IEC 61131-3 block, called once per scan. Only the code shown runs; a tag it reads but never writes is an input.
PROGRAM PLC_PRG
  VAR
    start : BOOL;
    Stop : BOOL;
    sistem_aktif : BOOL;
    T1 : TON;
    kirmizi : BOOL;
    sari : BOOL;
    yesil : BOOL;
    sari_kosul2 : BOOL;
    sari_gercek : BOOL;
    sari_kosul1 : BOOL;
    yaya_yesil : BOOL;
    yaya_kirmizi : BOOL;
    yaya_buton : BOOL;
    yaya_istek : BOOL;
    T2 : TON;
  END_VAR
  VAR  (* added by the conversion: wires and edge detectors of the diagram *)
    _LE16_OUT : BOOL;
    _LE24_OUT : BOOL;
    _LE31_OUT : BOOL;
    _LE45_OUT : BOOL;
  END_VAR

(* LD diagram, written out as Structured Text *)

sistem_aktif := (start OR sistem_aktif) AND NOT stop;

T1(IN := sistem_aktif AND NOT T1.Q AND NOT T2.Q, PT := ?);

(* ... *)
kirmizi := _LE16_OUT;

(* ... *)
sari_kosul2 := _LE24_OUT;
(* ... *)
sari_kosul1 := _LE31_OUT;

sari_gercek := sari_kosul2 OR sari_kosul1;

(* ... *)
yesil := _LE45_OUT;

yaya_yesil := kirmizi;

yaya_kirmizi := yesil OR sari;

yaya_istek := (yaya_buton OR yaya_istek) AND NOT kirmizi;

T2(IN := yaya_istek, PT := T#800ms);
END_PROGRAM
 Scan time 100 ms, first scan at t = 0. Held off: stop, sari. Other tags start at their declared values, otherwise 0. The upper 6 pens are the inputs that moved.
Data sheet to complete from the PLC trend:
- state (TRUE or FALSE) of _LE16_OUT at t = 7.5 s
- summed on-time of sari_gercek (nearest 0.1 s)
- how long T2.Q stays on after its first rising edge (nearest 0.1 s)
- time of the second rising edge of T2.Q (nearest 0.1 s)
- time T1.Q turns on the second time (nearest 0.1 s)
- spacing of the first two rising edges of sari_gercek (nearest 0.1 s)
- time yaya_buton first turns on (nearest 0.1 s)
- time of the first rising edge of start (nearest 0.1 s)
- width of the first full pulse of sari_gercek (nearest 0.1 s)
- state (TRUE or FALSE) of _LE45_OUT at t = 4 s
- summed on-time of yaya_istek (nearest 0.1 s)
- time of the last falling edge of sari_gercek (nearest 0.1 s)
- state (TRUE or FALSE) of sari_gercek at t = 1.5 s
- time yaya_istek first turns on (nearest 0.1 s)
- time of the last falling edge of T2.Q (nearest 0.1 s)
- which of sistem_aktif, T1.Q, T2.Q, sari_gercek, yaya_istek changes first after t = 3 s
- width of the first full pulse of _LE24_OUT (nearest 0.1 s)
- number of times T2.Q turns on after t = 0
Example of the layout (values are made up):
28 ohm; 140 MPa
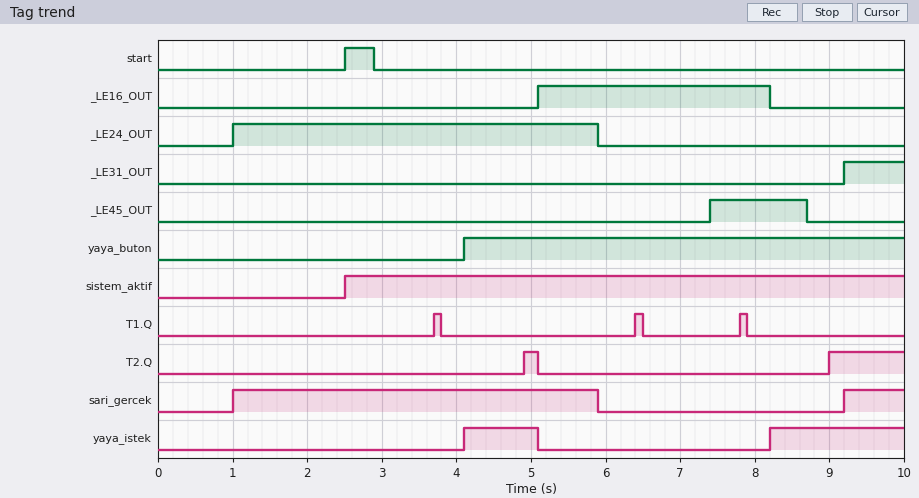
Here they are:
TRUE; 5.7 s; 0.2 s; 9.0 s; 6.4 s; 8.2 s; 4.1 s; 2.5 s; 4.9 s; FALSE; 2.8 s; 5.9 s; TRUE; 4.1 s; 5.1 s; T1.Q; 4.9 s; 2
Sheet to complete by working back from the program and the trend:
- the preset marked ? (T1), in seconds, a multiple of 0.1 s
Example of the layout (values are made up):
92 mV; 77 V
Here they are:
1.2 s
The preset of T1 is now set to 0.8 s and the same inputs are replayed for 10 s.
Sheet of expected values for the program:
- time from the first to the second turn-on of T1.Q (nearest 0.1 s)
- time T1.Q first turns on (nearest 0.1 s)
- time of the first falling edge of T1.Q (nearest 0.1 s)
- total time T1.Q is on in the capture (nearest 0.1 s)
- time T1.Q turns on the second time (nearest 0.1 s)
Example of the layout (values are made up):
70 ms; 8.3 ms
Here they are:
1.0 s; 3.3 s; 3.4 s; 0.6 s; 4.3 s
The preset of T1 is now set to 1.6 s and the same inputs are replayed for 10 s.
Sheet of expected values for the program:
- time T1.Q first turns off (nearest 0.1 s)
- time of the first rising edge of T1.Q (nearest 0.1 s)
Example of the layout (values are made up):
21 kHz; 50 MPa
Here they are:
4.2 s; 4.1 s
